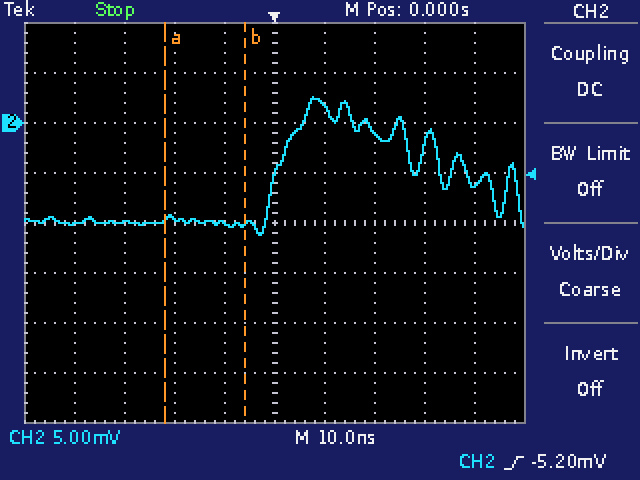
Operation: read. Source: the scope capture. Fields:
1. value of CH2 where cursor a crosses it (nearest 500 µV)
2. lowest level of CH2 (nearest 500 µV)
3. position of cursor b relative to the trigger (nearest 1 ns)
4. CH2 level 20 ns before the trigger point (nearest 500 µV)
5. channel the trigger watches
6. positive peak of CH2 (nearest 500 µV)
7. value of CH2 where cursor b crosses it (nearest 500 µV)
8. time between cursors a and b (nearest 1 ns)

-9.5 mV
-11.0 mV
-6 ns
-9.5 mV
CH2
2.5 mV
-10.0 mV
16 ns
